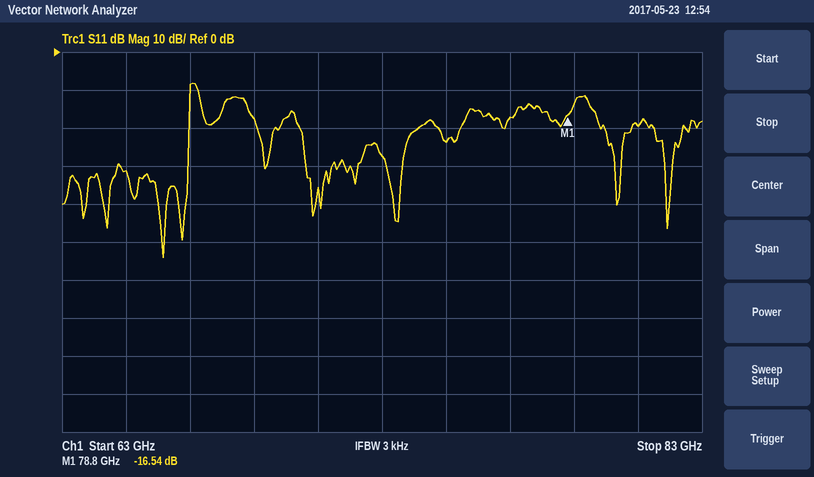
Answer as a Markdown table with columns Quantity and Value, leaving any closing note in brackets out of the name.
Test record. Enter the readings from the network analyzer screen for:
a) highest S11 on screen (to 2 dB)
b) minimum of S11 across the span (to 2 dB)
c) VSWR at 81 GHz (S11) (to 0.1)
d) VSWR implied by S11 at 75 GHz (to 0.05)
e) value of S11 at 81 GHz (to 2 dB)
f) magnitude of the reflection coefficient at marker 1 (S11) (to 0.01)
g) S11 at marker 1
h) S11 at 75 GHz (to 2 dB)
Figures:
| Quantity | Value |
|---|---|
| highest S11 on screen | -8 dB |
| minimum of S11 across the span | -54 dB |
| VSWR at 81 GHz (S11) | 1.2 |
| VSWR implied by S11 at 75 GHz | 1.15 |
| value of S11 at 81 GHz | -20 dB |
| magnitude of the reflection coefficient at marker 1 (S11) | 0.15 |
| S11 at marker 1 | -16.54 dB |
| S11 at 75 GHz | -24 dB |
